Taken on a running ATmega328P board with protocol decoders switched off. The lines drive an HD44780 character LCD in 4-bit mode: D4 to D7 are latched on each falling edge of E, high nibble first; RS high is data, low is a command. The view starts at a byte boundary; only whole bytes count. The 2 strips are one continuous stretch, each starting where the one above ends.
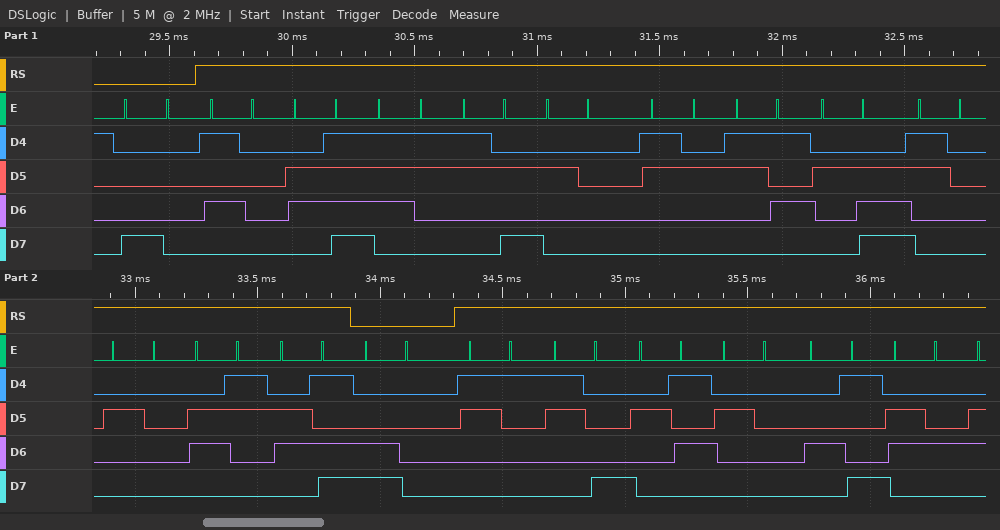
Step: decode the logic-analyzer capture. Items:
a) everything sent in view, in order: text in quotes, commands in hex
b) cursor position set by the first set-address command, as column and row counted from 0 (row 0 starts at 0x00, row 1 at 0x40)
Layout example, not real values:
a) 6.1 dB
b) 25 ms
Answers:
a) 0x80 "Pos: 25.0 cm" 0xC0 "18% Id"
b) column 0, row 0
